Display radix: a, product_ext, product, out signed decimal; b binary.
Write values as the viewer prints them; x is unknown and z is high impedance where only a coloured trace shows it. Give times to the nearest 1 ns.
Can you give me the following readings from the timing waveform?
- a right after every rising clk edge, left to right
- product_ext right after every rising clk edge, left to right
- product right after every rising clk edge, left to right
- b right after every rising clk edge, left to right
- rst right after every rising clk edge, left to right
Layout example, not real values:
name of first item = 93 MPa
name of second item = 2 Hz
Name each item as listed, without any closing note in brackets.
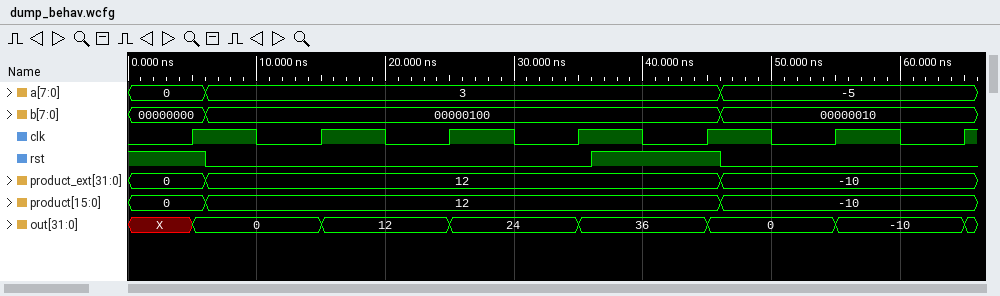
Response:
a right after every rising clk edge, left to right = 0, 3, 3, 3, 3, -5, -5
product_ext right after every rising clk edge, left to right = 0, 12, 12, 12, 12, -10, -10
product right after every rising clk edge, left to right = 0, 12, 12, 12, 12, -10, -10
b right after every rising clk edge, left to right = 00000000, 00000100, 00000100, 00000100, 00000100, 00000010, 00000010
rst right after every rising clk edge, left to right = 1 0 0 0 1 0 0
